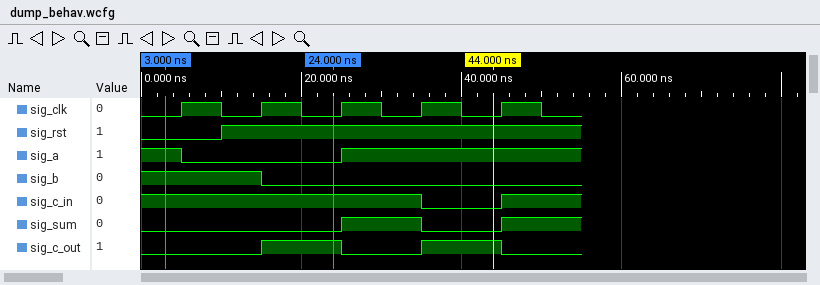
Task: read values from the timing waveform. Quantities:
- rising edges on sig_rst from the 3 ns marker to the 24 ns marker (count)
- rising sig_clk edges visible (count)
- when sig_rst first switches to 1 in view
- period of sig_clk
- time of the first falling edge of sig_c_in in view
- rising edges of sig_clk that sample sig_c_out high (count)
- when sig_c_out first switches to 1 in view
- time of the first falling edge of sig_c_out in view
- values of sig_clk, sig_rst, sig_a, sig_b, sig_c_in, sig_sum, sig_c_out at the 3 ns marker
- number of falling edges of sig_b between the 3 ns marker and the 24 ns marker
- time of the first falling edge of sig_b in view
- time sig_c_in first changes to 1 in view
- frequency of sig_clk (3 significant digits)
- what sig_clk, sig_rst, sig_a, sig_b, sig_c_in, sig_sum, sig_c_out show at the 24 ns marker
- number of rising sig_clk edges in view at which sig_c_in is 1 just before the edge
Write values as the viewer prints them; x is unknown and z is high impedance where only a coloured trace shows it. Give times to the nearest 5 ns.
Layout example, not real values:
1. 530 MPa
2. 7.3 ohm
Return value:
1. 1
2. 5
3. 10 ns
4. 10 ns
5. 35 ns
6. 2
7. 15 ns
8. 25 ns
9. sig_clk=0, sig_rst=0, sig_a=1, sig_b=1, sig_c_in=1, sig_sum=0, sig_c_out=0
10. 1
11. 15 ns
12. 45 ns
13. 100 MHz
14. sig_clk=0, sig_rst=1, sig_a=0, sig_b=0, sig_c_in=1, sig_sum=0, sig_c_out=1
15. 4
